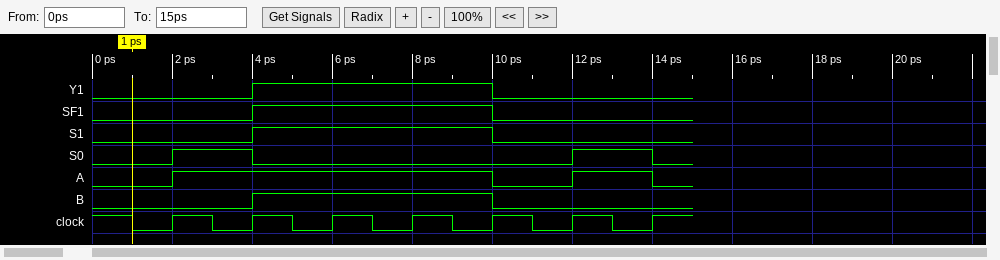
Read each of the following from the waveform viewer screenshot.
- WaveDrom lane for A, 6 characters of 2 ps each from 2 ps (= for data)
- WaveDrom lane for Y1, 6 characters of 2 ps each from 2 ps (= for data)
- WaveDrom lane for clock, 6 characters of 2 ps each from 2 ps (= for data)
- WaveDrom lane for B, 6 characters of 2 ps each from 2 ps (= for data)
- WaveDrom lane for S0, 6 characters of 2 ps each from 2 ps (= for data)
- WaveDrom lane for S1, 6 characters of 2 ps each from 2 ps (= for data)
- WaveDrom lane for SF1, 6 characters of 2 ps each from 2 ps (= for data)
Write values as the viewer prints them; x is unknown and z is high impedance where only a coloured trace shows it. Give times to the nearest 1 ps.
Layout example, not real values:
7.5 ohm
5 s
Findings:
{name: 'A', wave: '1...01'}
{name: 'Y1', wave: '01..0.'}
{name: 'clock', wave: 'p.....'}
{name: 'B', wave: '01..0.'}
{name: 'S0', wave: '10...1'}
{name: 'S1', wave: '01..0.'}
{name: 'SF1', wave: '01..0.'}
